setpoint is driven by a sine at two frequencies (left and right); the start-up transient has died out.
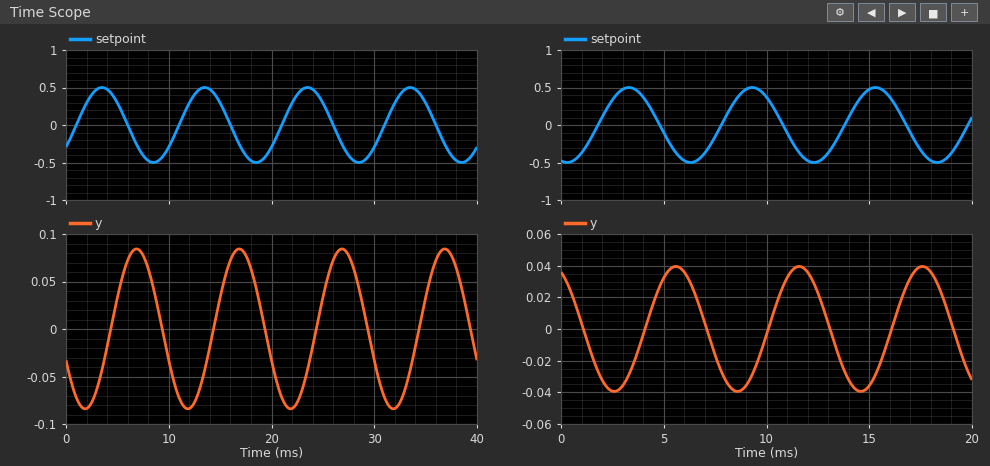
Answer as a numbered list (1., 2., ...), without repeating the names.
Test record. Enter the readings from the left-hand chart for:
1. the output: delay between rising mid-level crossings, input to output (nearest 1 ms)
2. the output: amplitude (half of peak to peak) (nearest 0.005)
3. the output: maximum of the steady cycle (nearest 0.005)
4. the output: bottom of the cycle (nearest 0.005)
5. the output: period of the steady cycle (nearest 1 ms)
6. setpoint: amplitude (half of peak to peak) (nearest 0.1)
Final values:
1. 3 ms
2. 0.085
3. 0.085
4. -0.085
5. 10 ms
6. 0.5
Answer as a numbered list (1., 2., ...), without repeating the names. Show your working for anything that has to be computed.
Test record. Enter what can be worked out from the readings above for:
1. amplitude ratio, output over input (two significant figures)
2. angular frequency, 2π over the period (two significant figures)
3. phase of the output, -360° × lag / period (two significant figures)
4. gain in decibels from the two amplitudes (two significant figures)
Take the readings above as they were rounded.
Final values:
1. 0.085 / 0.5 = 0.17
2. 2π / 10 = 0.63 rad/ms
3. -360 × 3 / 10 = -110°
4. 20 log10(0.085 / 0.5) = -15 dB
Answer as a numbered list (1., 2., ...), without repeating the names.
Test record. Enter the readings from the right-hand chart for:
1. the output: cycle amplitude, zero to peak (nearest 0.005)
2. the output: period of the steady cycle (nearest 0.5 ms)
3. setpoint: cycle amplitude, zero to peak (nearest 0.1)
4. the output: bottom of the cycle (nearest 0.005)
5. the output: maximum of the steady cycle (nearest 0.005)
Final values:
1. 0.040
2. 6.0 ms
3. 0.5
4. -0.040
5. 0.040
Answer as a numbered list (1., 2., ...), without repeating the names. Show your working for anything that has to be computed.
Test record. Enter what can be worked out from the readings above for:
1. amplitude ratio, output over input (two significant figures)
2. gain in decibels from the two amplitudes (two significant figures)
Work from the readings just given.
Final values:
1. 0.04 / 0.5 = 0.080
2. 20 log10(0.04 / 0.5) = -22 dB
